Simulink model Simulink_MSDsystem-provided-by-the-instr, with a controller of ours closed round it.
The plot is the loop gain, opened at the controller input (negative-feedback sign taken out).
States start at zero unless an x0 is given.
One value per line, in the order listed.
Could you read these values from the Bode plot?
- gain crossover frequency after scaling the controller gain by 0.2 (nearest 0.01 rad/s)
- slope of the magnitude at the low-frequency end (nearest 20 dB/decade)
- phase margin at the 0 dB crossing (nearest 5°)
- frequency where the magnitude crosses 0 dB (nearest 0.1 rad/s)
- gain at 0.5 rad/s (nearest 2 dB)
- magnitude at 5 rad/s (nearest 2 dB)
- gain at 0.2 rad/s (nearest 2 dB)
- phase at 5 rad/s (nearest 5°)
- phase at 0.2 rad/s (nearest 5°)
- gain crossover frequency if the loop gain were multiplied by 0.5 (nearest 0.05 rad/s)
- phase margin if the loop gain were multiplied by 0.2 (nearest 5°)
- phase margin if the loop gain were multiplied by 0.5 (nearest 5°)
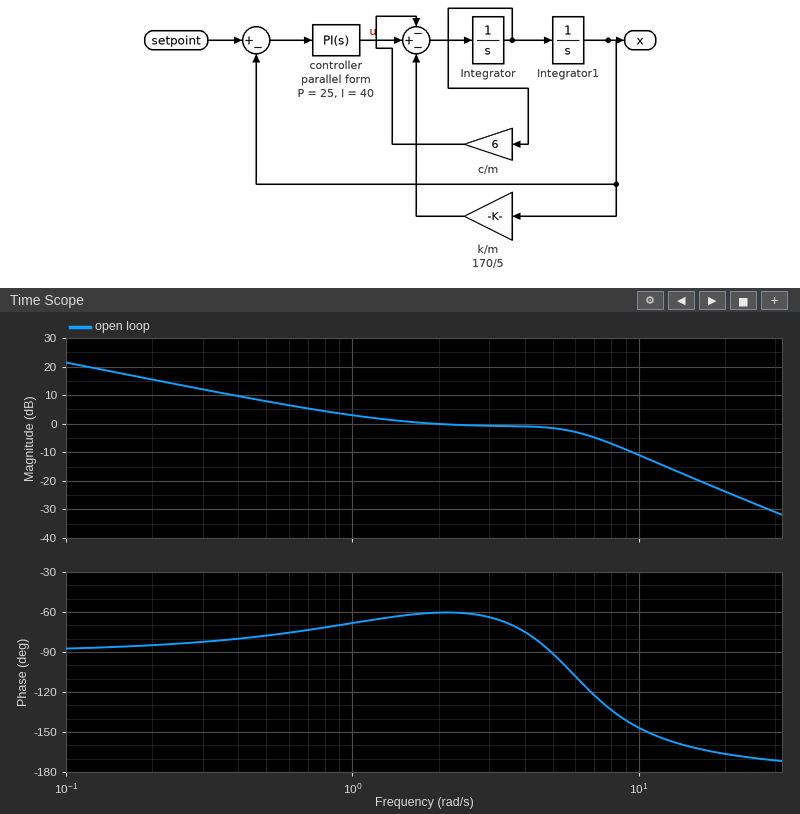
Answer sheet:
0.24 rad/s
-20 dB/decade
120°
1.9 rad/s
8 dB
-2 dB
16 dB
-90°
-85°
0.65 rad/s
95°
105°
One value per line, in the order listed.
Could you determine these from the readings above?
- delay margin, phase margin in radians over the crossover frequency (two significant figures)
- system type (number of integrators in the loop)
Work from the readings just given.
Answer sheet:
1.1 s
1
